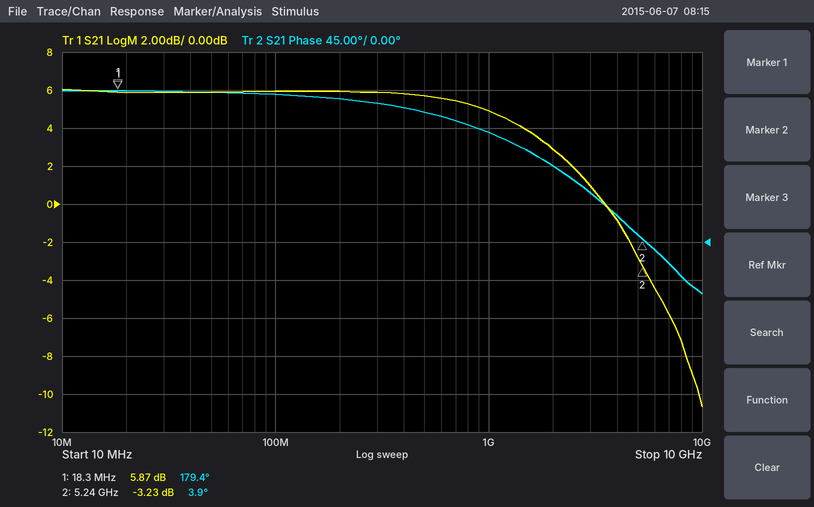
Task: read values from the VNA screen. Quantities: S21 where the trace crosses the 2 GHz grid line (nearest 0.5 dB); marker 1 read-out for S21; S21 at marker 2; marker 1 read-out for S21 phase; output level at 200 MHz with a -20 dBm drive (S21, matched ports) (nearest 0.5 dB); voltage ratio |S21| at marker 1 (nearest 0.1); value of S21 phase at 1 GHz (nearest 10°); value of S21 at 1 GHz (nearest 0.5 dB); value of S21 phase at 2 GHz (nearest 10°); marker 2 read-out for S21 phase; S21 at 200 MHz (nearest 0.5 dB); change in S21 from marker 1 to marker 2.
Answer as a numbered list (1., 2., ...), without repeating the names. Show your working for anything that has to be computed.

1. 3.0 dB
2. 5.87 dB
3. -3.23 dB
4. 179.4°
5. -20 dBm + (6.0 dB) = -14.0 dBm
6. 10^(5.87/20) ≈ 2.0
7. 130°
8. 5.0 dB
9. 90°
10. 3.9°
11. 6.0 dB
12. -3.23 − (5.87) = -9.10 dB
